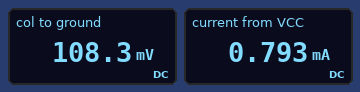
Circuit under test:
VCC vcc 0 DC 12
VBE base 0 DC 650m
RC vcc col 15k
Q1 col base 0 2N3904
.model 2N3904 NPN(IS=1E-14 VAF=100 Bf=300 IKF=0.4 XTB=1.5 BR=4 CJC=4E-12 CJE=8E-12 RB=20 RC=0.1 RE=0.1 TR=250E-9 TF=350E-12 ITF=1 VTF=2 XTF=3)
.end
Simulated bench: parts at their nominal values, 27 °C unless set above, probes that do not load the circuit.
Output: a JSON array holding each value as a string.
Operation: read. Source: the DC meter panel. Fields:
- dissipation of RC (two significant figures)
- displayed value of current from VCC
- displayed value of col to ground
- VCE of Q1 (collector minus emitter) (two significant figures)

["9.4 mW", "0.793 mA", "108.3 mV", "110 mV"]
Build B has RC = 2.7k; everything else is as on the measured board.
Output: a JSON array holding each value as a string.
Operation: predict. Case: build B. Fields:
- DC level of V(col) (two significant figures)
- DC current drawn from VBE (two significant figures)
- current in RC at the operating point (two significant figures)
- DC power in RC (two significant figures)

["9.6 V", "2.7 µA", "890 µA", "2.1 mW"]
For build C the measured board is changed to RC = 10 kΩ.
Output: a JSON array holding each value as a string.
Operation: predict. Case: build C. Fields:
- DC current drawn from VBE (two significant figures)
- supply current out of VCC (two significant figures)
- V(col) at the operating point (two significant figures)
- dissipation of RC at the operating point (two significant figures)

["2.7 µA", "840 µA", "3.6 V", "7.0 mW"]
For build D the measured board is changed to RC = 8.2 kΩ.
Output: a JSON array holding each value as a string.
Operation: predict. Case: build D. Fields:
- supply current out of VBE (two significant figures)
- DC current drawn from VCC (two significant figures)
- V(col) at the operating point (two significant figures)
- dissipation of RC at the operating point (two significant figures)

["2.7 µA", "850 µA", "5.0 V", "5.9 mW"]
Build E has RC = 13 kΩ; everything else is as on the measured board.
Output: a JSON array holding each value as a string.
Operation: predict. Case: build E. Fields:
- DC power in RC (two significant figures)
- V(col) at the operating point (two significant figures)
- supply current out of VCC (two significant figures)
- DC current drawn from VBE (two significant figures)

["8.7 mW", "1.3 V", "820 µA", "2.7 µA"]
